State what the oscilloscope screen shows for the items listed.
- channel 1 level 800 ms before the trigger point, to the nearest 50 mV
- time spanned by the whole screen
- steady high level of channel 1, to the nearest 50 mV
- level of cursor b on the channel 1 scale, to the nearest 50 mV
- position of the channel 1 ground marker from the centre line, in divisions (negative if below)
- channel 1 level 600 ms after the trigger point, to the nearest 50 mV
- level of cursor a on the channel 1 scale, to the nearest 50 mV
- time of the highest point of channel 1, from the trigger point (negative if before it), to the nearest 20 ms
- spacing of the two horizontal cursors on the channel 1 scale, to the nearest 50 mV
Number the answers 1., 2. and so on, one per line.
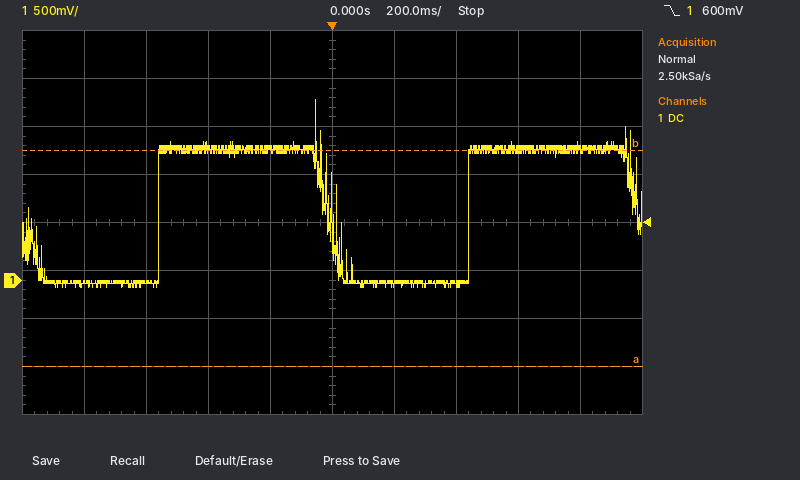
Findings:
1. -50 mV
2. 2 s
3. 1.35 V
4. 1.35 V
5. -1.2 div
6. 1.35 V
7. -900 mV
8. -60 ms
9. 2.25 V
